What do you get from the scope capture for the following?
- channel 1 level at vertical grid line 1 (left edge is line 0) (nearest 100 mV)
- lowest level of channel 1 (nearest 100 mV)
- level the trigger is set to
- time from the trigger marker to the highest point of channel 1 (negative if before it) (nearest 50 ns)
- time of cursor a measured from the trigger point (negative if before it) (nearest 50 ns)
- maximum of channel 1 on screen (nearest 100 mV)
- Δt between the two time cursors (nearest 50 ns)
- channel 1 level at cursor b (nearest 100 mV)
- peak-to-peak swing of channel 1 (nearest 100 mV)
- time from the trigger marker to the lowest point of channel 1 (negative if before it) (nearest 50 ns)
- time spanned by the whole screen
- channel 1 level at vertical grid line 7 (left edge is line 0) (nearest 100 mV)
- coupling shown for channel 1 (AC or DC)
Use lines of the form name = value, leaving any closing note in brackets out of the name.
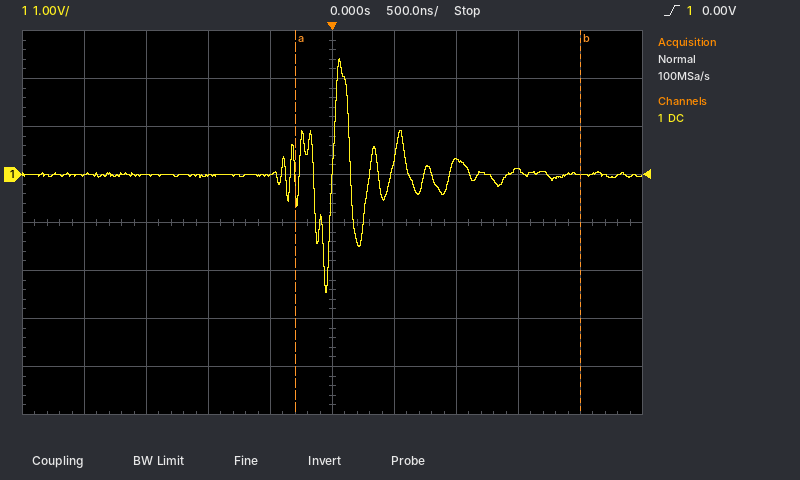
channel 1 level at vertical grid line 1 (left edge is line 0) = 0.0 V
lowest level of channel 1 = -2.5 V
level the trigger is set to = 0.00 V
time from the trigger marker to the highest point of channel 1 (negative if before it) = +50 ns
time of cursor a measured from the trigger point (negative if before it) = -300 ns
maximum of channel 1 on screen = 2.4 V
Δt between the two time cursors = 2.30 µs
channel 1 level at cursor b = 0.0 V
peak-to-peak swing of channel 1 = 4.9 V
time from the trigger marker to the lowest point of channel 1 (negative if before it) = -50 ns
time spanned by the whole screen = 5 µs
channel 1 level at vertical grid line 7 (left edge is line 0) = 300 mV
coupling shown for channel 1 = DC
